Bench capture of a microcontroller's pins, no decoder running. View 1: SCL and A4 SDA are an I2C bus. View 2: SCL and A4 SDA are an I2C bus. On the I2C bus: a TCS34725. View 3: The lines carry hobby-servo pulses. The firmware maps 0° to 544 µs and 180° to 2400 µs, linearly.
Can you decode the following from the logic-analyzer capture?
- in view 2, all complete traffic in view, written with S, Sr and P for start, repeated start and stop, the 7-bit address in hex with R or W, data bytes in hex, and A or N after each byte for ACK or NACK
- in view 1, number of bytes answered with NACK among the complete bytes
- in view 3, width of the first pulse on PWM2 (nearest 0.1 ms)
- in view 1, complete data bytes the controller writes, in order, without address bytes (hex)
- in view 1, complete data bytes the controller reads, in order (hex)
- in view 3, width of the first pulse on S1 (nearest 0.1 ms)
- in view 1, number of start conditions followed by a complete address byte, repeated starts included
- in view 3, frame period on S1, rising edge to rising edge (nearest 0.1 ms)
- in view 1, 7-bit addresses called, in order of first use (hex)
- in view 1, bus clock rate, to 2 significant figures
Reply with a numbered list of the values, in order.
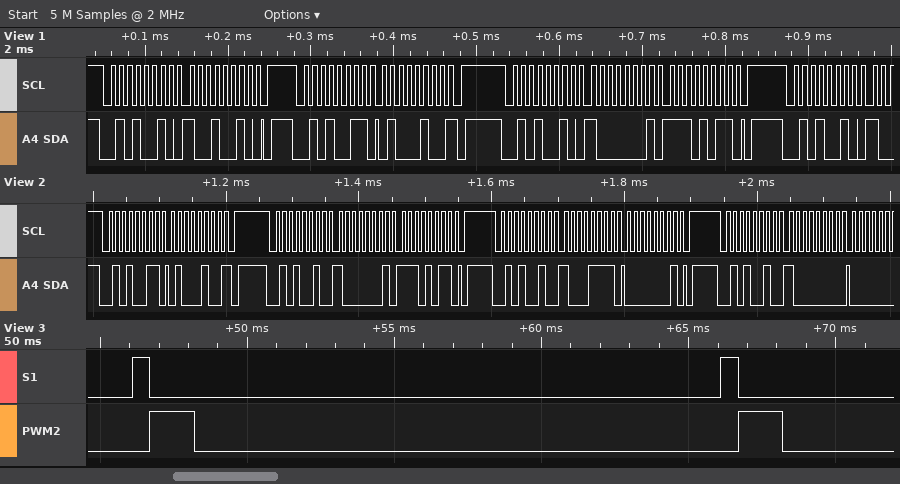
1. S 29R A 44 N P S 29W A 81 A EB A P S 29W A 8F A 01 A P S 29W A 80 A
2. 1
3. 1.5 ms
4. 92 81 EB
5. 44
6. 0.6 ms
7. 4
8. 20.0 ms
9. 0x29
10. 100 kHz
